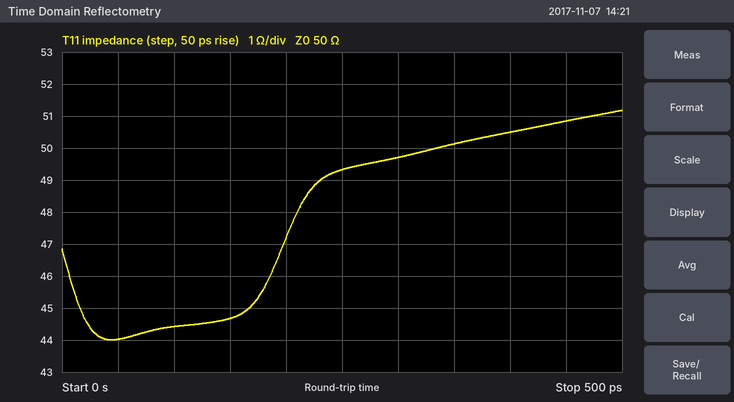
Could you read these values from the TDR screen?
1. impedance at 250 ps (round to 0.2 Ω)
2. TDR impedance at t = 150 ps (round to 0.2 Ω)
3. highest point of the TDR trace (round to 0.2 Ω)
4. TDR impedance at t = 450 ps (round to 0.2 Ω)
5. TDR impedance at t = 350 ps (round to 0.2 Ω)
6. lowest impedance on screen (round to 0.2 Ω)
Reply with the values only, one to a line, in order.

49.4 Ω
44.6 Ω
51.2 Ω
50.8 Ω
50.2 Ω
44.0 Ω
